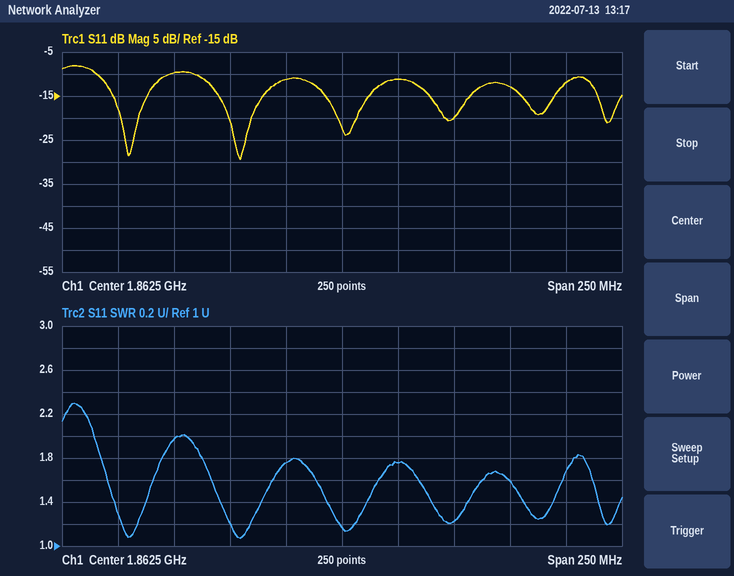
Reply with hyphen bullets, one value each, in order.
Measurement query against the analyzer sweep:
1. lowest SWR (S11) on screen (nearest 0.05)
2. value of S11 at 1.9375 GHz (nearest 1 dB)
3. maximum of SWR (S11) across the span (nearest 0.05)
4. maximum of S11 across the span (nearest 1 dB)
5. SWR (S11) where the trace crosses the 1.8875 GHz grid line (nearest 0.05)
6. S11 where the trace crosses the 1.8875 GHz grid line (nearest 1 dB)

- 1.05
- -13 dB
- 2.30
- -8 dB
- 1.75
- -11 dB
